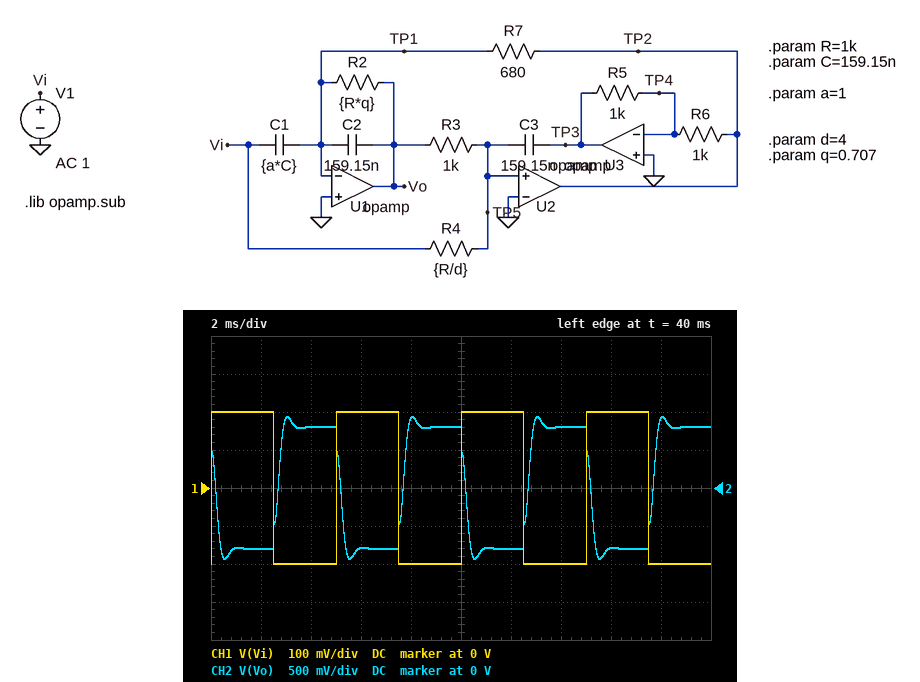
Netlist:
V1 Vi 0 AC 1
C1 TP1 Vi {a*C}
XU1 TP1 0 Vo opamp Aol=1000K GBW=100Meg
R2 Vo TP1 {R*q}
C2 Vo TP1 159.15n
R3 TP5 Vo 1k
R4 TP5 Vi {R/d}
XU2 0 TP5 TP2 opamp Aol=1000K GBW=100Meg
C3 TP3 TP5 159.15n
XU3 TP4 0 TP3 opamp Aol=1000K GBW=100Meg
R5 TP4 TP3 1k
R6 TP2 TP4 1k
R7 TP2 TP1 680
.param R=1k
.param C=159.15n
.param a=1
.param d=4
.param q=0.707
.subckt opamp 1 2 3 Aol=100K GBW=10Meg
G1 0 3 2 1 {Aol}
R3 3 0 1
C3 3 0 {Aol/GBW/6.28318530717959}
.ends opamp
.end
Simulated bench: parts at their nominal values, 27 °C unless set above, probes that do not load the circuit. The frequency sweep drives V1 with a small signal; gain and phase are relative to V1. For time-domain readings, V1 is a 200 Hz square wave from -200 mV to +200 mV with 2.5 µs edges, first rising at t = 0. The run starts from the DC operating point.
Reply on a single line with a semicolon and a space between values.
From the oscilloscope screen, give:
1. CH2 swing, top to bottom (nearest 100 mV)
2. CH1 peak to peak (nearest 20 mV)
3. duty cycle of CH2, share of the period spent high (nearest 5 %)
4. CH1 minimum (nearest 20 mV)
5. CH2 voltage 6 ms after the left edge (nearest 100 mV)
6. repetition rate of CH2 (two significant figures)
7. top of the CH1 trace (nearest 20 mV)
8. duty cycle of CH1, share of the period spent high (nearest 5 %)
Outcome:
1.9 V; 400 mV; 50 %; -200 mV; -800 mV; 200 Hz; 200 mV; 50 %
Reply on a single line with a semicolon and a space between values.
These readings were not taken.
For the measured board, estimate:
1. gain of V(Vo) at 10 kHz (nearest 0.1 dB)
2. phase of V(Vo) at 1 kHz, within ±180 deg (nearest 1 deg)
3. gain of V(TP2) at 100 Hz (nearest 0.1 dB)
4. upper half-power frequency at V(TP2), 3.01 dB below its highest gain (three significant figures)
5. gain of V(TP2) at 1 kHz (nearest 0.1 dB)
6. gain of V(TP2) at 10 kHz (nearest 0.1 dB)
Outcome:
-0.5 dB; 108 deg; 11.7 dB; 1.54 kHz; 12.7 dB; -10.3 dB
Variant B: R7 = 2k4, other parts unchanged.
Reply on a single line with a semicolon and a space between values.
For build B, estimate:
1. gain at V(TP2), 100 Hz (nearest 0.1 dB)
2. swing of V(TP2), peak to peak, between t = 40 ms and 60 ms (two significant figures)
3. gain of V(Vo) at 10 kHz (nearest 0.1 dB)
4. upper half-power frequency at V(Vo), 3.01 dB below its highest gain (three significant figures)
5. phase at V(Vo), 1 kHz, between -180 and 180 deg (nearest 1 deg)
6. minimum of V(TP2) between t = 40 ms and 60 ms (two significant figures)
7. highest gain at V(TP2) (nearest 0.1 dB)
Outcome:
22.4 dB; 5.4 V; -0.2 dB; 322 Hz; 68 deg; -2.7 V; 22.7 dB
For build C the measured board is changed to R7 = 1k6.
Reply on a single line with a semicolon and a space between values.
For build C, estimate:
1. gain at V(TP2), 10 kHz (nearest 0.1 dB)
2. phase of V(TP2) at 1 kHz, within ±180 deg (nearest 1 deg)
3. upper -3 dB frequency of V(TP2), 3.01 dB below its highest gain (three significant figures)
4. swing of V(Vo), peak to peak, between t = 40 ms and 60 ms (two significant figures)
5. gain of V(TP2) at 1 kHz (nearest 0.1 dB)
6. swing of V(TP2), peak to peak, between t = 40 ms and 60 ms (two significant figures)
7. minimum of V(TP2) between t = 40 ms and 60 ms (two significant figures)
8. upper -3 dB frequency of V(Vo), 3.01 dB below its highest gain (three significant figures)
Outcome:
-10.3 dB; -77 deg; 643 Hz; 1.6 V; 12.8 dB; 3.6 V; -1.8 V; 496 Hz
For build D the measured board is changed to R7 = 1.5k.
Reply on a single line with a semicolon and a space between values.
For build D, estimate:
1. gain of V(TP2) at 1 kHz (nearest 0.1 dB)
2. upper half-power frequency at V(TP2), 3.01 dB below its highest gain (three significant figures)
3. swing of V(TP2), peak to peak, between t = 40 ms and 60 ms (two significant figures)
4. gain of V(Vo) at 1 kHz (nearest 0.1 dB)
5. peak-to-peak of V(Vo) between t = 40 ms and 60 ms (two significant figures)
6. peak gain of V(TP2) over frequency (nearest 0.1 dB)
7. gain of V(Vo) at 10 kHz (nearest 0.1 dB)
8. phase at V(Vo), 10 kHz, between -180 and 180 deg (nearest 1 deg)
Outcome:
12.9 dB; 700 Hz; 3.4 V; 1.2 dB; 1.6 V; 18.6 dB; -0.3 dB; -172 deg
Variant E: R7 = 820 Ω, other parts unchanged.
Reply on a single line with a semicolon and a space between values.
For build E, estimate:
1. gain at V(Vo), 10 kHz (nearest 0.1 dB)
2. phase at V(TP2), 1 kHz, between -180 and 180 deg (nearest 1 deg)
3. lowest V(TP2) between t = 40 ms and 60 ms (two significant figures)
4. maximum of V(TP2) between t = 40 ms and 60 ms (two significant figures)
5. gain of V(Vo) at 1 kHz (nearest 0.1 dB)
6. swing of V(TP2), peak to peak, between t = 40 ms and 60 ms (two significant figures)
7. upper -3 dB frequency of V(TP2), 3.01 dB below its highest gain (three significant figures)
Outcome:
-0.4 dB; -53 deg; -1.1 V; 1.1 V; 8.7 dB; 2.2 V; 1.35 kHz
